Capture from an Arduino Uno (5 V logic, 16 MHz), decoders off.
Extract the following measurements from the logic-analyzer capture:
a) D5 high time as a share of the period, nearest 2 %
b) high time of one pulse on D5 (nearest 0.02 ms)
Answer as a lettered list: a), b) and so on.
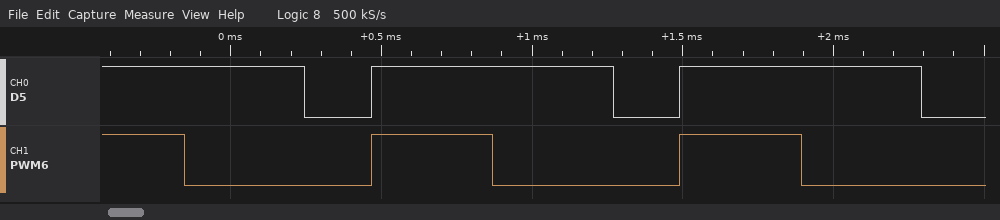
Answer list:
a) 78 %
b) 0.80 ms
